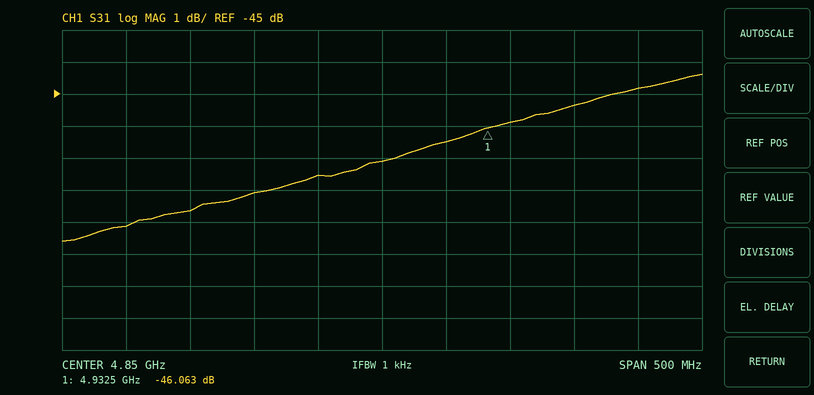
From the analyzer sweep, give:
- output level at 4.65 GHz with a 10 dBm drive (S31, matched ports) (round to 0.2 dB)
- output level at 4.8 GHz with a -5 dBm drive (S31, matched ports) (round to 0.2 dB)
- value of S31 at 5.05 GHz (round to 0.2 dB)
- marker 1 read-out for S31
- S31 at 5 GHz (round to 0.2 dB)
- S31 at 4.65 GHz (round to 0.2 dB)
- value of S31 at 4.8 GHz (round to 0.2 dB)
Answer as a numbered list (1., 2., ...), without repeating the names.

1. -39.2 dBm
2. -52.6 dBm
3. -44.8 dB
4. -46.063 dB
5. -45.4 dB
6. -49.2 dB
7. -47.6 dB
